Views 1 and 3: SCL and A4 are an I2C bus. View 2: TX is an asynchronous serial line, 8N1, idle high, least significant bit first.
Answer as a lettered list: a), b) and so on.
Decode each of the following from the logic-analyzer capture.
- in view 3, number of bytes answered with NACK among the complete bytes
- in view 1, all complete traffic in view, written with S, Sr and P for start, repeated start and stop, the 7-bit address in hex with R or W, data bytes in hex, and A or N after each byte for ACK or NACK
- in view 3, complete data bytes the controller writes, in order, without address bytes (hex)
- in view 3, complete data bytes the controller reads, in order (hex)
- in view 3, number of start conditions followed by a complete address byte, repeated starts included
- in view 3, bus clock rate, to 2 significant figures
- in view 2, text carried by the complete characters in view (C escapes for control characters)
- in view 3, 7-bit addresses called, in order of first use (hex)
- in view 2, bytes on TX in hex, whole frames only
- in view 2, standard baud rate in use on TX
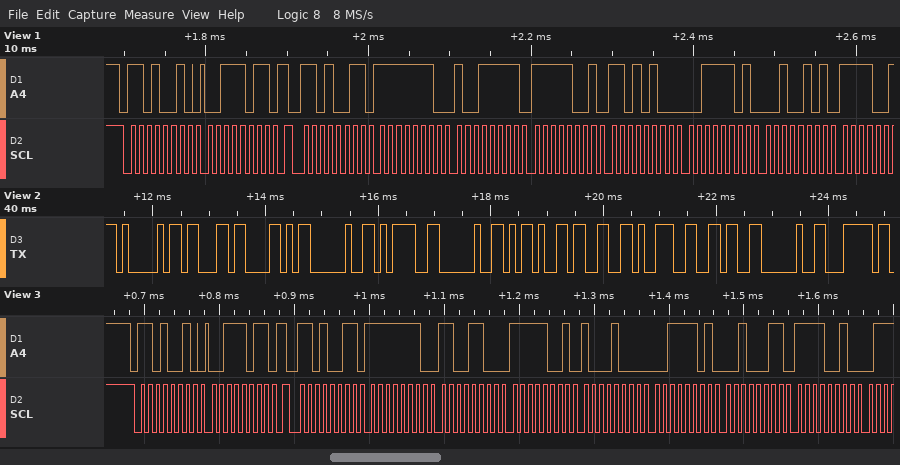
a) 0
b) S 69W A 3B A Sr 69R A FE A 9F A F9 A D4 A 3D A 25 A
c) 3B
d) FE CC F9 88 3D 23 F2
e) 2
f) 100 kHz
g) "AcX = -396 |"
h) 0x69
i) 0x41 0x63 0x58 0x20 0x3D 0x20 0x2D 0x33 0x39 0x36 0x20 0x7C
j) 9600 baud
